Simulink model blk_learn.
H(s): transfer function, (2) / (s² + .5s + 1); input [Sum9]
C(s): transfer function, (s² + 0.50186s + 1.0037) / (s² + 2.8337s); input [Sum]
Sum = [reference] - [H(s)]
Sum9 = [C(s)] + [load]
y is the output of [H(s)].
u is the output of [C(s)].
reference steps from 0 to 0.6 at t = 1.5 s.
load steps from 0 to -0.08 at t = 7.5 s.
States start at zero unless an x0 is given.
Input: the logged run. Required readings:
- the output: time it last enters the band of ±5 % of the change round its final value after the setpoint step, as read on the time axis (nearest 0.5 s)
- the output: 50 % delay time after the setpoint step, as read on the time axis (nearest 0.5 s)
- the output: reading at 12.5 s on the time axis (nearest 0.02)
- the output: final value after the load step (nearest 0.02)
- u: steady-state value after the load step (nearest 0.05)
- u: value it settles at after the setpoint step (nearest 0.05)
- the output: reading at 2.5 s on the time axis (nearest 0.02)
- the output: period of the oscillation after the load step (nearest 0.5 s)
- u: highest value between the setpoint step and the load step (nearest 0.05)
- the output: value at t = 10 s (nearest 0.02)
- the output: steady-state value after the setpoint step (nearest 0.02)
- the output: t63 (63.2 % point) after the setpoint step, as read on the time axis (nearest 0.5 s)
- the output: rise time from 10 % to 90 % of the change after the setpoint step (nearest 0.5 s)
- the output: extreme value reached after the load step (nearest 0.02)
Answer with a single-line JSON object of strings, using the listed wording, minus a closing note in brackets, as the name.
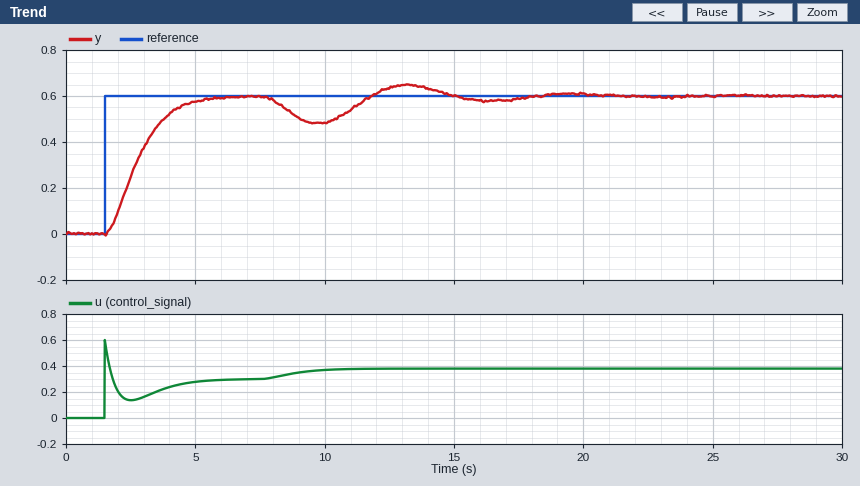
{"the output: time it last enters the band of ±5 % of the change round its final value after the setpoint step, as read on the time axis": "5.0 s", "the output: 50 % delay time after the setpoint step, as read on the time axis": "2.5 s", "the output: reading at 12.5 s on the time axis": "0.64", "the output: final value after the load step": "0.60", "u: steady-state value after the load step": "0.40", "u: value it settles at after the setpoint step": "0.30", "the output: reading at 2.5 s on the time axis": "0.24", "the output: period of the oscillation after the load step": "6.5 s", "u: highest value between the setpoint step and the load step": "0.60", "the output: value at t = 10 s": "0.48", "the output: steady-state value after the setpoint step": "0.60", "the output: t63 (63.2 % point) after the setpoint step, as read on the time axis": "3.0 s", "the output: rise time from 10 % to 90 % of the change after the setpoint step": "2.5 s", "the output: extreme value reached after the load step": "0.48"}
